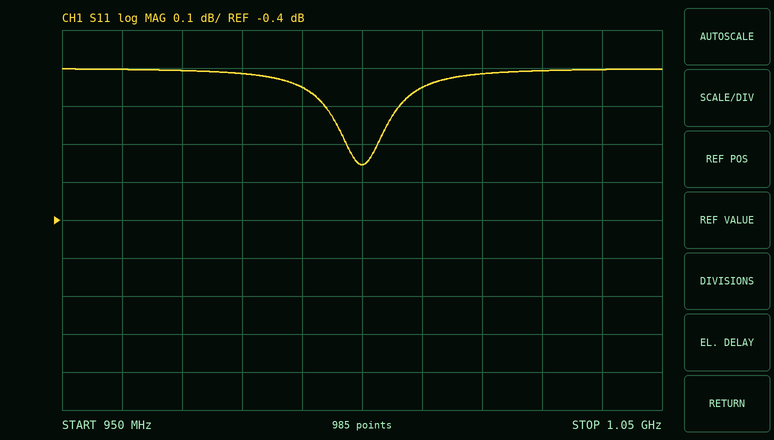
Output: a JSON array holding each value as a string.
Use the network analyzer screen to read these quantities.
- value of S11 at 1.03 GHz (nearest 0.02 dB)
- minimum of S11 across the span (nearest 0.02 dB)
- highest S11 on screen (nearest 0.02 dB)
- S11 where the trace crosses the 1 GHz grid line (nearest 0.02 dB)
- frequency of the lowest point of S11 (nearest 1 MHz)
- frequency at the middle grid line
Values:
["0.00 dB", "-0.26 dB", "0.00 dB", "-0.26 dB", "1.000 GHz", "1 GHz"]
